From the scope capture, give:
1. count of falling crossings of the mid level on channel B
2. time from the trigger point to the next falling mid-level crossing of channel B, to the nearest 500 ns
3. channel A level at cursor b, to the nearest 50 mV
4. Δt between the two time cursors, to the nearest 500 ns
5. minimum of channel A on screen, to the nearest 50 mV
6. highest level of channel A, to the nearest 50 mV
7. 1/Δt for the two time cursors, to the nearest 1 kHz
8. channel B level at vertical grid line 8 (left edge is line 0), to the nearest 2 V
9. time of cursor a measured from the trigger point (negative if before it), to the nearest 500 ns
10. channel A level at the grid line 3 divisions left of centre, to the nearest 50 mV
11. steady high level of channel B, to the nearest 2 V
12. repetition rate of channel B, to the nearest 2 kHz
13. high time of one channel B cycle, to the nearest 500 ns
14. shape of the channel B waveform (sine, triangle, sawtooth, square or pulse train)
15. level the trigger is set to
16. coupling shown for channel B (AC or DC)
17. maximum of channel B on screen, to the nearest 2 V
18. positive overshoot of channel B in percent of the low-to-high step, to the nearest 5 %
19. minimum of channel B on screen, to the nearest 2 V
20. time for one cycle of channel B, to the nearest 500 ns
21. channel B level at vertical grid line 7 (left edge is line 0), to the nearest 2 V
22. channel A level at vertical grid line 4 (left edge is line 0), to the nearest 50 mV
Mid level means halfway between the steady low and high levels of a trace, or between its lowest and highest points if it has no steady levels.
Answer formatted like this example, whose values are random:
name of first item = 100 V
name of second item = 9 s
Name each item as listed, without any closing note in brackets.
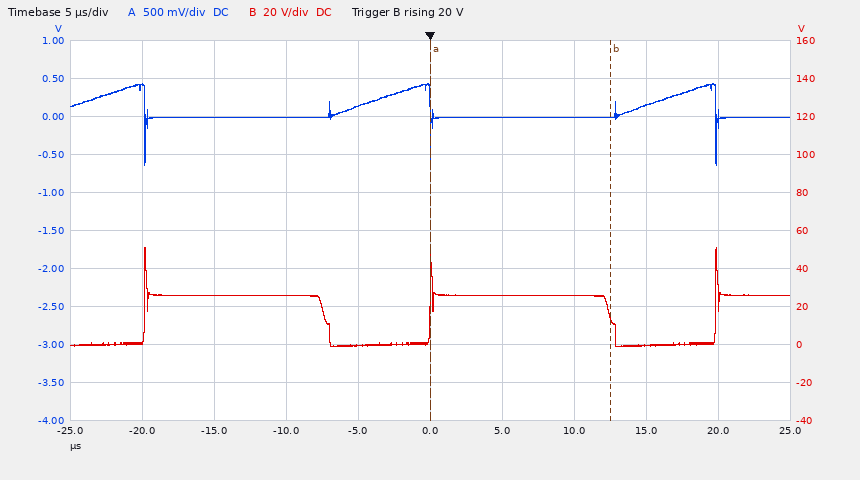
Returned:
count of falling crossings of the mid level on channel B = 2
time from the trigger point to the next falling mid-level crossing of channel B, to the nearest 500 ns = 12.5 µs
channel A level at cursor b, to the nearest 50 mV = 0 mV
Δt between the two time cursors, to the nearest 500 ns = 12.5 µs
minimum of channel A on screen, to the nearest 50 mV = -650 mV
highest level of channel A, to the nearest 50 mV = 450 mV
1/Δt for the two time cursors, to the nearest 1 kHz = 80 kHz
channel B level at vertical grid line 8 (left edge is line 0), to the nearest 2 V = 0 V
time of cursor a measured from the trigger point (negative if before it), to the nearest 500 ns = 0.0 µs
channel A level at the grid line 3 divisions left of centre, to the nearest 50 mV = 0 mV
steady high level of channel B, to the nearest 2 V = 26 V
repetition rate of channel B, to the nearest 2 kHz = 50 kHz
high time of one channel B cycle, to the nearest 500 ns = 12.5 µs
shape of the channel B waveform = pulse train
level the trigger is set to = 20 V
coupling shown for channel B = DC
maximum of channel B on screen, to the nearest 2 V = 52 V
positive overshoot of channel B in percent of the low-to-high step, to the nearest 5 % = 95 %
minimum of channel B on screen, to the nearest 2 V = -2 V
time for one cycle of channel B, to the nearest 500 ns = 20.0 µs
channel B level at vertical grid line 7 (left edge is line 0), to the nearest 2 V = 26 V
channel A level at vertical grid line 4 (left edge is line 0), to the nearest 50 mV = 150 mV
